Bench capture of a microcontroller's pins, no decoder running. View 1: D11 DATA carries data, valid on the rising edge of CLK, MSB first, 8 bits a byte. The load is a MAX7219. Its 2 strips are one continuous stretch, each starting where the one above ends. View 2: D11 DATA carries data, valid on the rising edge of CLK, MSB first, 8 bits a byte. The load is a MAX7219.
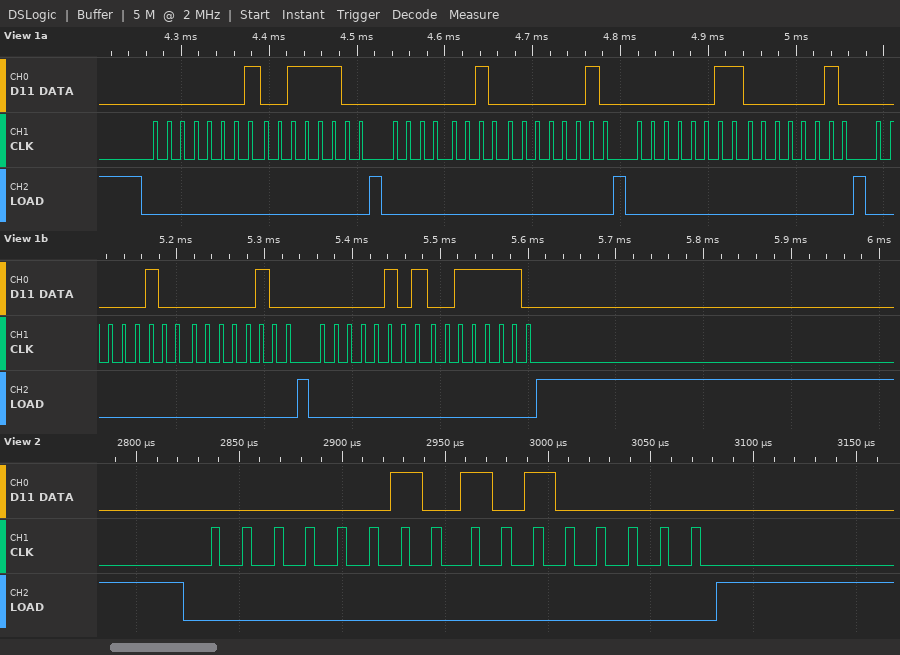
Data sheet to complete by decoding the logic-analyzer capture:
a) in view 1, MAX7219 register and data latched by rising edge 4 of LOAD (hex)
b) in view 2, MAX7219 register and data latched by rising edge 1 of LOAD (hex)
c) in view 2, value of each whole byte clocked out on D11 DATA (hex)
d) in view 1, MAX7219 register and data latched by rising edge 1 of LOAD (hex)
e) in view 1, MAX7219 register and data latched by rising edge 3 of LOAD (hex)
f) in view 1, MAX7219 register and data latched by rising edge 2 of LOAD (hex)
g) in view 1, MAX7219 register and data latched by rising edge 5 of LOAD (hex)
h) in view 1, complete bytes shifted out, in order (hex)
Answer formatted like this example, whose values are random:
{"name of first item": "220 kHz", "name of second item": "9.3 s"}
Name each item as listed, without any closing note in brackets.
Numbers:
{"in view 1, MAX7219 register and data latched by rising edge 4 of LOAD": "register 0x4, data 0x04", "in view 2, MAX7219 register and data latched by rising edge 1 of LOAD": "register 0x2, data 0xA0", "in view 2, value of each whole byte clocked out on D11 DATA": "02 A0", "in view 1, MAX7219 register and data latched by rising edge 1 of LOAD": "register 0x1, data 0x3C", "in view 1, MAX7219 register and data latched by rising edge 3 of LOAD": "register 0x3, data 0x02", "in view 1, MAX7219 register and data latched by rising edge 2 of LOAD": "register 0x2, data 0x02", "in view 1, MAX7219 register and data latched by rising edge 5 of LOAD": "register 0x5, data 0x3E", "in view 1, complete bytes shifted out, in order": "01 3C 02 02 03 02 04 04 05 3E"}
